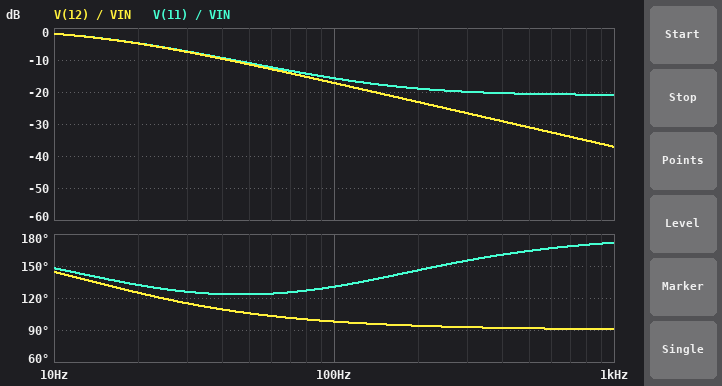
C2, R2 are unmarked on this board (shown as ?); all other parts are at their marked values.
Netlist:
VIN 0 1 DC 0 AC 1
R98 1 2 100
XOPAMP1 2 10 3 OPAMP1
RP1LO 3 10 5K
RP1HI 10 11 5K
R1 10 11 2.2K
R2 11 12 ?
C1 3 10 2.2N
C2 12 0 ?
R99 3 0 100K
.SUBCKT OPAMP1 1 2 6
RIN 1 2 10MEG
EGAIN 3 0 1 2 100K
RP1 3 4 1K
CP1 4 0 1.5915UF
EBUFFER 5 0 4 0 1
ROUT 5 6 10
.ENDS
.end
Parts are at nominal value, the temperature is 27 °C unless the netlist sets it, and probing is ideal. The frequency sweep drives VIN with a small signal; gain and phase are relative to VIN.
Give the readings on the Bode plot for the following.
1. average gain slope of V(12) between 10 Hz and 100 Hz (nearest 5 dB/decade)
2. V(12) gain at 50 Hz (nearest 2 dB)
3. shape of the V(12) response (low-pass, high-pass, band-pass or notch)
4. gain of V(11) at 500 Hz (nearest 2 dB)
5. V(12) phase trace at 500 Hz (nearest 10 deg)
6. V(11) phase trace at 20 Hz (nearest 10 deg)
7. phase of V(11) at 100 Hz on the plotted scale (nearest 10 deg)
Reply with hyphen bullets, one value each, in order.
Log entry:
- -15 dB/decade
- -12 dB
- low-pass
- -20 dB
- 90 deg
- 130 deg
- 130 deg
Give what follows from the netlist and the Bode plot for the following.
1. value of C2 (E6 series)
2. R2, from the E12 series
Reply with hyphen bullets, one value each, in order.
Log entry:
- 6.8 µF
- 150 Ω
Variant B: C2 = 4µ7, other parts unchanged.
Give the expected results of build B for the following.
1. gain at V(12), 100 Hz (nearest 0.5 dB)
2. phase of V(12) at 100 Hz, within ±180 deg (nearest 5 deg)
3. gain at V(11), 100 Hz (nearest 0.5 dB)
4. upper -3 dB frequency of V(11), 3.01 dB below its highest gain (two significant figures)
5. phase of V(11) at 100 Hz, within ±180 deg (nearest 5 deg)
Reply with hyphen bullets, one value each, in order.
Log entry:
- -14.0 dB
- 100 deg
- -13.5 dB
- 20 Hz
- 125 deg
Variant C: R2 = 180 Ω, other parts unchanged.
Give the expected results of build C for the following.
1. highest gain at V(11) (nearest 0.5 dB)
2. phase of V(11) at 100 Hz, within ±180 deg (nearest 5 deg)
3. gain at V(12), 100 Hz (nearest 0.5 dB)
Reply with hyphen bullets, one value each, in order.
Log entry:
- 0 dB
- 135 deg
- -17.5 dB
